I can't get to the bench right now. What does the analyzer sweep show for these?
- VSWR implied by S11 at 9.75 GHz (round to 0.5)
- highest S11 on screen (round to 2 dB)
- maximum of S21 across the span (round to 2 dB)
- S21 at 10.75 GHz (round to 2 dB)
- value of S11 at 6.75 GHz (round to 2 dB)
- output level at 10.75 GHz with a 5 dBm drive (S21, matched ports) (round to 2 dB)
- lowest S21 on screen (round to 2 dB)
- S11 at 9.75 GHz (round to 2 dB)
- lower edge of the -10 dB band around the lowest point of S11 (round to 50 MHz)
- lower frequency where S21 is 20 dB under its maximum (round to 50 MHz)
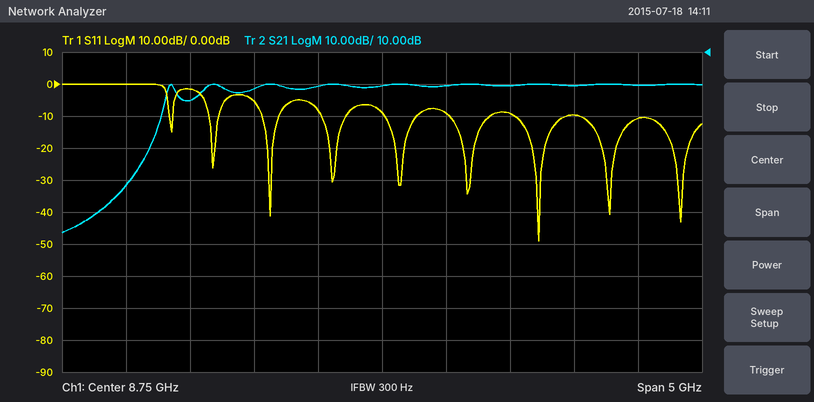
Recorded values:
2.0
0 dB
0 dB
0 dB
0 dB
4 dBm
-46 dB
-10 dB
9.80 GHz
6.95 GHz
